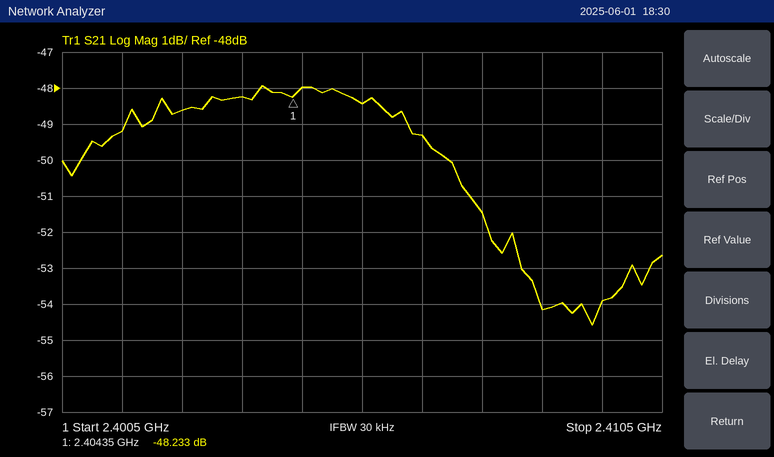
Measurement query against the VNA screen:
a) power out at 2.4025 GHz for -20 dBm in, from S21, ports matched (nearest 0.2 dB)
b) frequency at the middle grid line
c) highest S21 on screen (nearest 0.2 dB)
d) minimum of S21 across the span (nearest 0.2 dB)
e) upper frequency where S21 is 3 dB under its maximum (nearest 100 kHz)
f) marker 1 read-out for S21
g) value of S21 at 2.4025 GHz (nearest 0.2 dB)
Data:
-68.6 dBm
2.4055 GHz
-48.0 dB
-54.6 dB
2.4073 GHz
-48.233 dB
-48.6 dB
